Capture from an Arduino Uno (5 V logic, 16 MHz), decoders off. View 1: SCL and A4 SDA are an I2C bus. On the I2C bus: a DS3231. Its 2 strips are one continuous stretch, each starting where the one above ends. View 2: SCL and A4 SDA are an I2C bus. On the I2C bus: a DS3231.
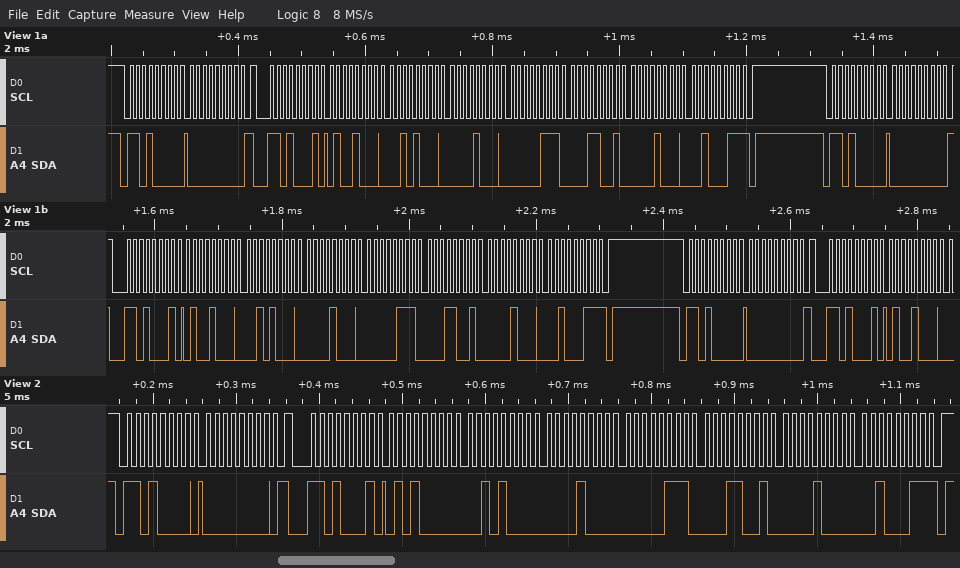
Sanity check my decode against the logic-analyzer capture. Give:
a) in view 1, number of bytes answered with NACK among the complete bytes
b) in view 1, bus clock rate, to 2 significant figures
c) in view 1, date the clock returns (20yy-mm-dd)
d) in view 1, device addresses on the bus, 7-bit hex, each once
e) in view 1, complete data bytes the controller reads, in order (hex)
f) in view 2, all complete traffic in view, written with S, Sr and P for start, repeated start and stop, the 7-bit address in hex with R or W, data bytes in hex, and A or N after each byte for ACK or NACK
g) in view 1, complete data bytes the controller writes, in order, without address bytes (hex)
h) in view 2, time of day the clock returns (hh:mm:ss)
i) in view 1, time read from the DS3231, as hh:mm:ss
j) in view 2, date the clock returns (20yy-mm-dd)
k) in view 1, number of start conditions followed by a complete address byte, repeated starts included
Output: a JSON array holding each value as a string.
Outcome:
["2", "100 kHz", "2023-08-19", "0x68", "48 28 08 07 19 08 23 48 28 08 07 19 08 23 48", "S 68W A 00 A Sr 68R A 50 A 28 A 08 A 07 A 19 A 08 A 23 N P", "00 00 00", "08:28:50", "08:28:48", "2023-08-19", "6"]
